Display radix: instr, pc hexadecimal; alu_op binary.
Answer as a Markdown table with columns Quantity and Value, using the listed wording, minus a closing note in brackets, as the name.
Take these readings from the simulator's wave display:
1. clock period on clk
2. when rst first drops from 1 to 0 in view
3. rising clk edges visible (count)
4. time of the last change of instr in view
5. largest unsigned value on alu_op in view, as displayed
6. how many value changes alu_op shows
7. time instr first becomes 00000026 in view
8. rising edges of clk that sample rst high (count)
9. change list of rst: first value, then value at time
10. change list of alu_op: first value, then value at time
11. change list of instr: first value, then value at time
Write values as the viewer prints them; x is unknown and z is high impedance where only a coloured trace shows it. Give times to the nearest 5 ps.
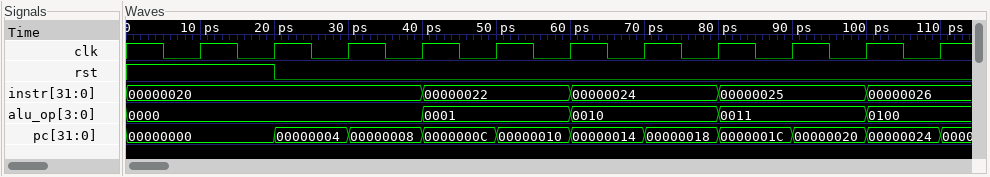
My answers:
| Quantity | Value |
|---|---|
| clock period on clk | 10 ps |
| when rst first drops from 1 to 0 in view | 20 ps |
| rising clk edges visible | 11 |
| time of the last change of instr in view | 100 ps |
| largest unsigned value on alu_op in view, as displayed | 0100 |
| how many value changes alu_op shows | 4 |
| time instr first becomes 00000026 in view | 100 ps |
| rising edges of clk that sample rst high | 2 |
| change list of rst: first value, then value at time | 1, 0 at 20 ps |
| change list of alu_op: first value, then value at time | 0000, 0001 at 40 ps, 0010 at 60 ps, 0011 at 80 ps, 0100 at 100 ps |
| change list of instr: first value, then value at time | 00000020, 00000022 at 40 ps, 00000024 at 60 ps, 00000025 at 80 ps, 00000026 at 100 ps |
